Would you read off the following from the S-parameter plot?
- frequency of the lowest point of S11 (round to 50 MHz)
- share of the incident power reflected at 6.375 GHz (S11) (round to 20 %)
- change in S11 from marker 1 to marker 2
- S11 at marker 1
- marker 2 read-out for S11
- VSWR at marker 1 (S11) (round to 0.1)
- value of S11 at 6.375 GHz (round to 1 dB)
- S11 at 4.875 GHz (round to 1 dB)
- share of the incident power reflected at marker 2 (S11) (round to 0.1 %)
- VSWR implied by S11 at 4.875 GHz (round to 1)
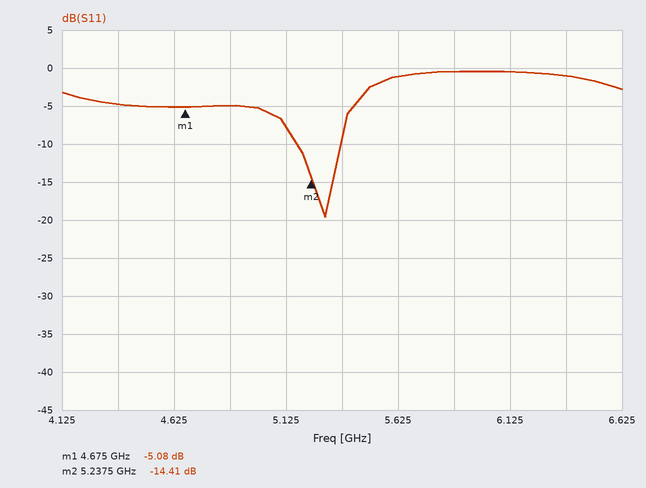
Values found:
5.30 GHz
80 %
-9.33 dB
-5.08 dB
-14.41 dB
3.5
-1 dB
-5 dB
3.6 %
4
